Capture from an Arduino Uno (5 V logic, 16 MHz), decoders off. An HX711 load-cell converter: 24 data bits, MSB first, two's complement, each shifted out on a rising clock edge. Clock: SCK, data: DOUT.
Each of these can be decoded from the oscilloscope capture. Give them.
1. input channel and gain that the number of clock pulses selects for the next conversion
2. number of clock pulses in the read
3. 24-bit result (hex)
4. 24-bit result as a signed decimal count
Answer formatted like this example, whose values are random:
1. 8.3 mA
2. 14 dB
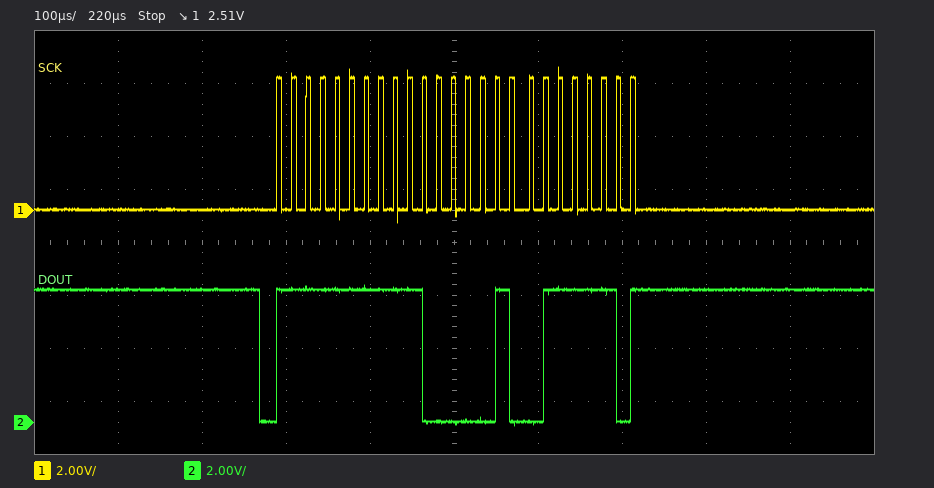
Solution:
1. channel A, gain 128
2. 25
3. 0xFFC13E
4. -16066
